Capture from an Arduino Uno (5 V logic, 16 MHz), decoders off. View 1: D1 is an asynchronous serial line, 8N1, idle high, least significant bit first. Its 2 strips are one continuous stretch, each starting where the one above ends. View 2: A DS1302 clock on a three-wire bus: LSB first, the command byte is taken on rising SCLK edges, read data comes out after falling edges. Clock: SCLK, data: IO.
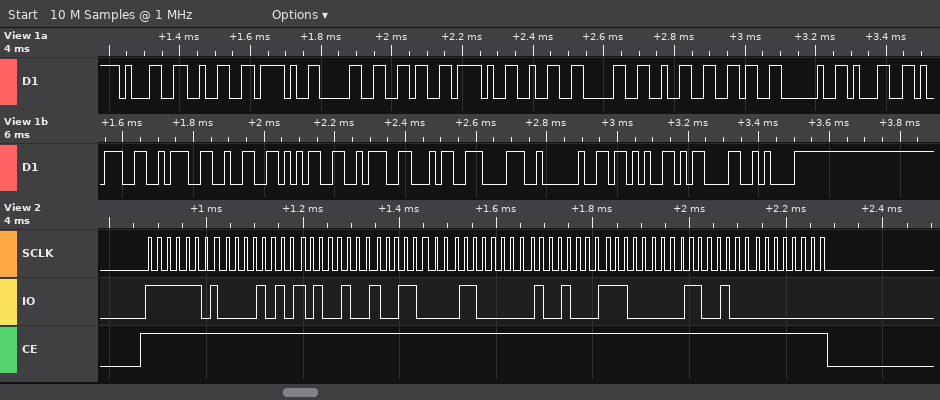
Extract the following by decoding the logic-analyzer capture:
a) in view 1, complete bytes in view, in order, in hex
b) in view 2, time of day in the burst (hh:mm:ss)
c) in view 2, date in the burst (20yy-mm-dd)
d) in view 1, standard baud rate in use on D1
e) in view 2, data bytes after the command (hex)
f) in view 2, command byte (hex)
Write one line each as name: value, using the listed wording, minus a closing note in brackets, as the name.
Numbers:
in view 1, complete bytes in view, in order, in hex: 31 32 2F 30 36 2F 32 30 32 36 20 31 39 3A 32 35 3A 34 38 20 2B 0D 0A
in view 2, time of day in the burst: 19:25:50
in view 2, date in the burst: 2026-12-06
in view 1, standard baud rate in use on D1: 57600 baud
in view 2, data bytes after the command: 50 25 19 06 12 07 26 00
in view 2, command byte: 0xBF
